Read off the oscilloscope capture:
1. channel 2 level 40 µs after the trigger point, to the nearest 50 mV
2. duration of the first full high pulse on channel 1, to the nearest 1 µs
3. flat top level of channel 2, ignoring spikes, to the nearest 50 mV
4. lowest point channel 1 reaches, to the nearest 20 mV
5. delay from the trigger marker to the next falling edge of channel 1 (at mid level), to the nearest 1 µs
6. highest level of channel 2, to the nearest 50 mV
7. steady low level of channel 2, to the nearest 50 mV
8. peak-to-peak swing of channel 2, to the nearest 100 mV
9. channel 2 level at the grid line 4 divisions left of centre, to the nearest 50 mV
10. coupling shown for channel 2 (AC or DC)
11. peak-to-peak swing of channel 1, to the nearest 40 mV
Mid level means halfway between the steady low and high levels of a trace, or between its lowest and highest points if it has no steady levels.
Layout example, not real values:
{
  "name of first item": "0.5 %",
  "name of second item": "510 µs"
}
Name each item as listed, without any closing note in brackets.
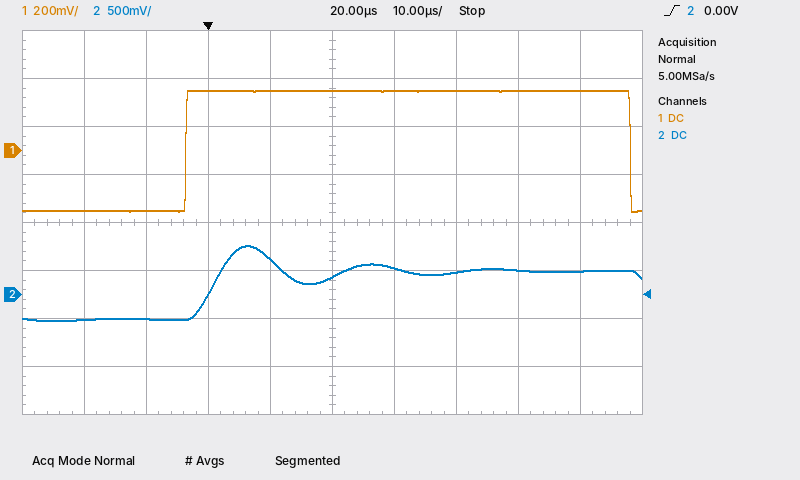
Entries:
{
  "channel 2 level 40 µs after the trigger point, to the nearest 50 mV": "250 mV",
  "duration of the first full high pulse on channel 1, to the nearest 1 µs": "72 µs",
  "flat top level of channel 2, ignoring spikes, to the nearest 50 mV": "250 mV",
  "lowest point channel 1 reaches, to the nearest 20 mV": "-260 mV",
  "delay from the trigger marker to the next falling edge of channel 1 (at mid level), to the nearest 1 µs": "68 µs",
  "highest level of channel 2, to the nearest 50 mV": "500 mV",
  "steady low level of channel 2, to the nearest 50 mV": "-250 mV",
  "peak-to-peak swing of channel 2, to the nearest 100 mV": "800 mV",
  "channel 2 level at the grid line 4 divisions left of centre, to the nearest 50 mV": "-250 mV",
  "coupling shown for channel 2": "DC",
  "peak-to-peak swing of channel 1, to the nearest 40 mV": "520 mV"
}
